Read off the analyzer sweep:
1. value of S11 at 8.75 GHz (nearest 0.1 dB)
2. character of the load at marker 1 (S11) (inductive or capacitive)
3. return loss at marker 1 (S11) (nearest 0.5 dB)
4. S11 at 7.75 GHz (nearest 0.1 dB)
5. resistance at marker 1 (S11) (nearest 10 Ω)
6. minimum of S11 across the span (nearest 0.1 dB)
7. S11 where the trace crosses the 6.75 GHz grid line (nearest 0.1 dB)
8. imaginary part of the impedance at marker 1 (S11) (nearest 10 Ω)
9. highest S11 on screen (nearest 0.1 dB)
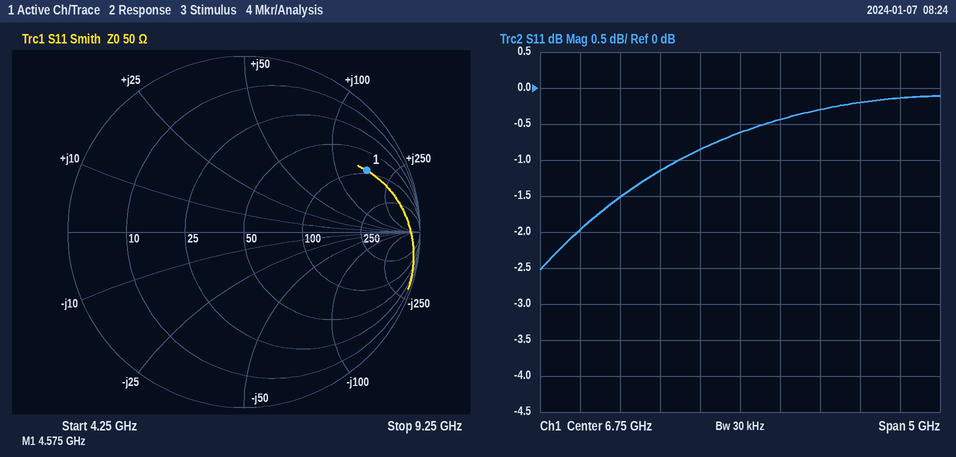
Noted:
-0.1 dB
inductive
2.0 dB
-0.3 dB
90 Ω
-2.5 dB
-0.6 dB
+160 Ω
-0.1 dB
